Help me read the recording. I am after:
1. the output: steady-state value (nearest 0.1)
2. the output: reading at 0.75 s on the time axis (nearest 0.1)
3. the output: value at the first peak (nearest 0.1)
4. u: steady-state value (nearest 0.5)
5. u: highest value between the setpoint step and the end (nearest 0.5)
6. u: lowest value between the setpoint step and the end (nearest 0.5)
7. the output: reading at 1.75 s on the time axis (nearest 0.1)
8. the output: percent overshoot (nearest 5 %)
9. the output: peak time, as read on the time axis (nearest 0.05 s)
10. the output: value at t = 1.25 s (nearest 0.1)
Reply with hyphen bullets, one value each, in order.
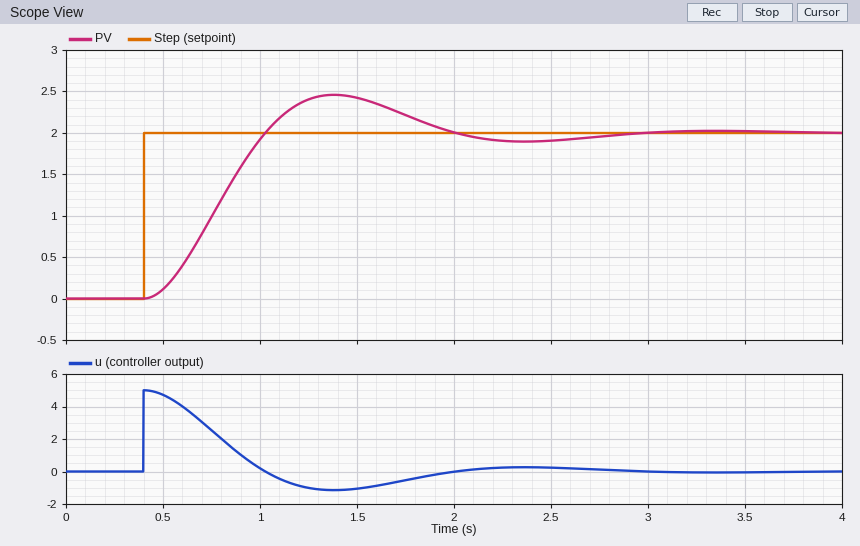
- 2.0
- 1.0
- 2.5
- 0.0
- 5.0
- -1.0
- 2.2
- 25 %
- 1.40 s
- 2.4
